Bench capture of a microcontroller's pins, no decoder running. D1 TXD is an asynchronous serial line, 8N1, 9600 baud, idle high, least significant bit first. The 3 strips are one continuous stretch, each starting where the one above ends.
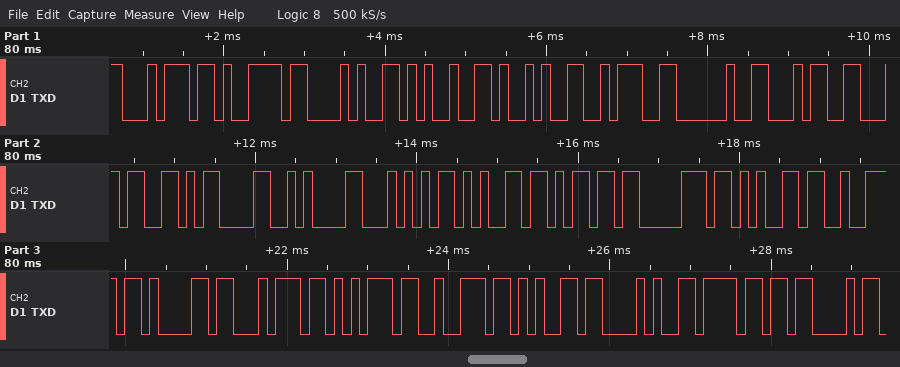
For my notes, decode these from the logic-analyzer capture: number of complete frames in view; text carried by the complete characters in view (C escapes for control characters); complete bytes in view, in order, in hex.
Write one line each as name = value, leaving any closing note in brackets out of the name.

number of complete frames in view = 25
text carried by the complete characters in view = "ty(%): 44\r\nTemperature(oC"
complete bytes in view, in order, in hex = 74 79 28 25 29 3A 20 34 34 0D 0A 54 65 6D 70 65 72 61 74 75 72 65 28 6F 43
